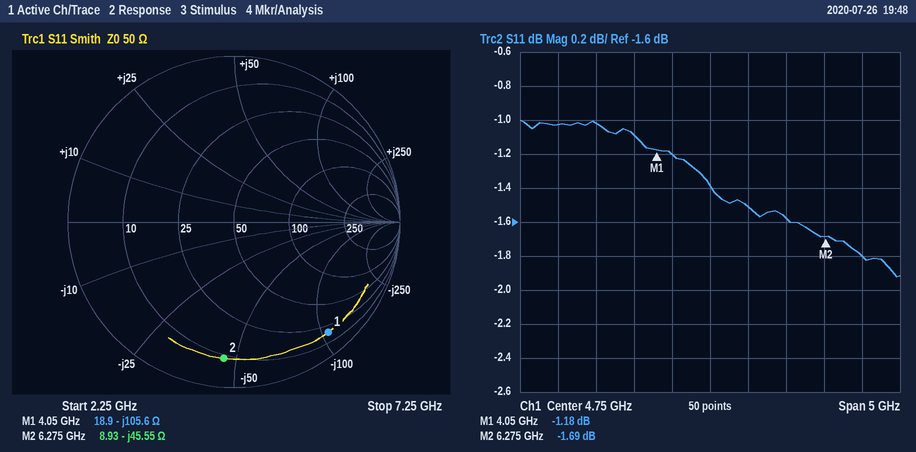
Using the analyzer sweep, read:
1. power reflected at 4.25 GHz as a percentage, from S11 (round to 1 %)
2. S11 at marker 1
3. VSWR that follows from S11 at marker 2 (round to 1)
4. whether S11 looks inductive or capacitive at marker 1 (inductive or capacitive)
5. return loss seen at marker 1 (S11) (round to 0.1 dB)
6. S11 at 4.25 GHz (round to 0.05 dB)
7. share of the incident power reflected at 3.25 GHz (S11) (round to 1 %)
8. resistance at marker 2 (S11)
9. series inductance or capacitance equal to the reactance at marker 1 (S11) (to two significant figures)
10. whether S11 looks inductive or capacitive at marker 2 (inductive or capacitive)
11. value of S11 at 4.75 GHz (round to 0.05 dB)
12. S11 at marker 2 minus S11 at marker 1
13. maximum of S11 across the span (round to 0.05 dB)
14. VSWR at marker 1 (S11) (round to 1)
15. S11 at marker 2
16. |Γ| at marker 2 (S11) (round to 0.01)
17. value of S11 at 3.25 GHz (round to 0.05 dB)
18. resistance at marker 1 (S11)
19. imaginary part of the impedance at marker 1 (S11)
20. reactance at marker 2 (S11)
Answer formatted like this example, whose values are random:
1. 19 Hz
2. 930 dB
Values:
1. 76 %
2. -1.18 dB
3. 10
4. capacitive
5. 1.2 dB
6. -1.20 dB
7. 79 %
8. 8.93 Ω
9. 370 fF
10. capacitive
11. -1.40 dB
12. -0.51 dB
13. -1.00 dB
14. 15
15. -1.69 dB
16. 0.82
17. -1.00 dB
18. 18.9 Ω
19. -105.6 Ω
20. -45.55 Ω
